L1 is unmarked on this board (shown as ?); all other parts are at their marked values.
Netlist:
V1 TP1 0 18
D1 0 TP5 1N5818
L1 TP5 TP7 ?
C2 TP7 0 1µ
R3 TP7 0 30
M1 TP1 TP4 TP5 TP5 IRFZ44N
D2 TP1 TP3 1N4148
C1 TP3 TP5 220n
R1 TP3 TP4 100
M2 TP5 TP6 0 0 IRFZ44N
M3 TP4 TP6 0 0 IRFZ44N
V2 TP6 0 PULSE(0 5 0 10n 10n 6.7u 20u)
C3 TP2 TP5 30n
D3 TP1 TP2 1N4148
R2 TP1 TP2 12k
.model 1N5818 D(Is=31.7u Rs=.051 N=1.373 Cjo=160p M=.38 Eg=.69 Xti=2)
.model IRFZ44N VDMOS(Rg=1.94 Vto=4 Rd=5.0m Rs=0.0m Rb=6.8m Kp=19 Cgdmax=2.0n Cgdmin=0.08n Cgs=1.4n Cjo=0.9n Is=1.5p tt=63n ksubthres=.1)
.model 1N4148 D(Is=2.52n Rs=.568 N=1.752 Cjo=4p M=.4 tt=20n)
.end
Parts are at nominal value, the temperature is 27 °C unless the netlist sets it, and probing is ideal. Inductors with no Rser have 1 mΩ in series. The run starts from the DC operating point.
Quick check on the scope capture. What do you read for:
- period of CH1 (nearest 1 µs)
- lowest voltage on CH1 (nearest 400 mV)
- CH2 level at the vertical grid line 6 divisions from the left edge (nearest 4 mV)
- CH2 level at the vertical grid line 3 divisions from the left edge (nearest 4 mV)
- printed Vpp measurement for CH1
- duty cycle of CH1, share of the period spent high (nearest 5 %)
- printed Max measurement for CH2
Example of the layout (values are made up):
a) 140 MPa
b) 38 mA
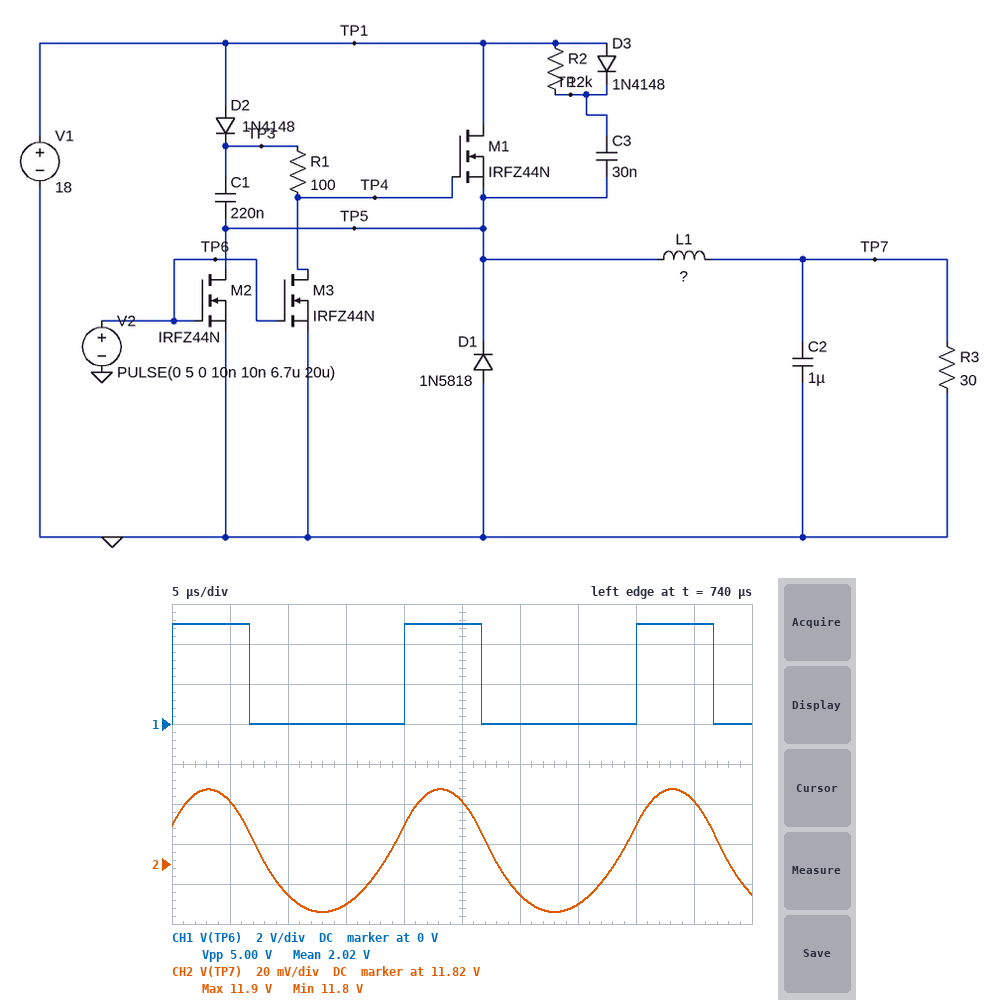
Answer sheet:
a) 20 µs
b) 0 V
c) 11.804 V
d) 11.800 V
e) 5.00 V
f) 35 %
g) 11.9 V
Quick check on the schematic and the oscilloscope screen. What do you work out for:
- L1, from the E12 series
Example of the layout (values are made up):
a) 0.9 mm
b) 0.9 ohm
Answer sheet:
a) 3.3 mH
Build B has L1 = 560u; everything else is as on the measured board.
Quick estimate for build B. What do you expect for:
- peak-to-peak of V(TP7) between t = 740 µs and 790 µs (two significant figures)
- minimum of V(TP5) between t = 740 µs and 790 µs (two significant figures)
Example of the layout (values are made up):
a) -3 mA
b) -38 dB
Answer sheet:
a) 370 mV
b) -360 mV
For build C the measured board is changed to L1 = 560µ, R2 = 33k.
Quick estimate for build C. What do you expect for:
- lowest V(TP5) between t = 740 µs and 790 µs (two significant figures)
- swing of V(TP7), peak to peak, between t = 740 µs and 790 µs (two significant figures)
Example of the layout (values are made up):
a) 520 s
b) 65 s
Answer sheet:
a) -360 mV
b) 370 mV
